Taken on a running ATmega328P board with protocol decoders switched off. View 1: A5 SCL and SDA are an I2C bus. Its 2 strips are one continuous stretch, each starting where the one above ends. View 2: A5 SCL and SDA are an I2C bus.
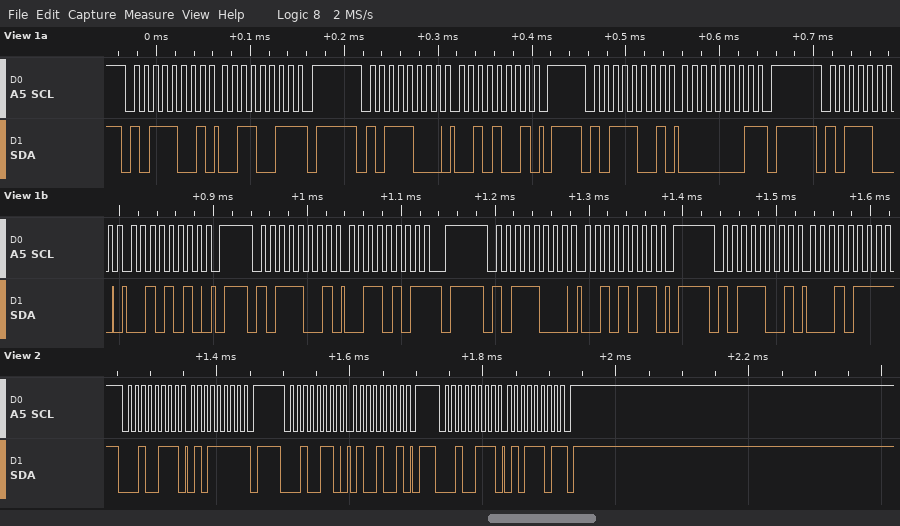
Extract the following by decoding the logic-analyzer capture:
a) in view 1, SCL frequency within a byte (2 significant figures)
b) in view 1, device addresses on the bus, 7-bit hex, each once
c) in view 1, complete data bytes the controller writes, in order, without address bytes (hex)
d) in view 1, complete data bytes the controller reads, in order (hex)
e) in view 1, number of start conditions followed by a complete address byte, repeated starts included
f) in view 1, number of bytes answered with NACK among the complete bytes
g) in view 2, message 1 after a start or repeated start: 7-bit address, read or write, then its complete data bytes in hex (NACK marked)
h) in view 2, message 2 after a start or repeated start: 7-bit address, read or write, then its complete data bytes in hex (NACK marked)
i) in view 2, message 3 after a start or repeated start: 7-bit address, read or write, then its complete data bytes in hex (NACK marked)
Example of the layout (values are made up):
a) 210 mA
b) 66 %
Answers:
a) 100 kHz
b) 0x5C
c) 29 2A 2B
d) 33 01 35 17
e) 7
f) 4
g) 0x13 read: 5F NACK
h) 0x13 write: 49
i) 0x13 read: 5D NACK
